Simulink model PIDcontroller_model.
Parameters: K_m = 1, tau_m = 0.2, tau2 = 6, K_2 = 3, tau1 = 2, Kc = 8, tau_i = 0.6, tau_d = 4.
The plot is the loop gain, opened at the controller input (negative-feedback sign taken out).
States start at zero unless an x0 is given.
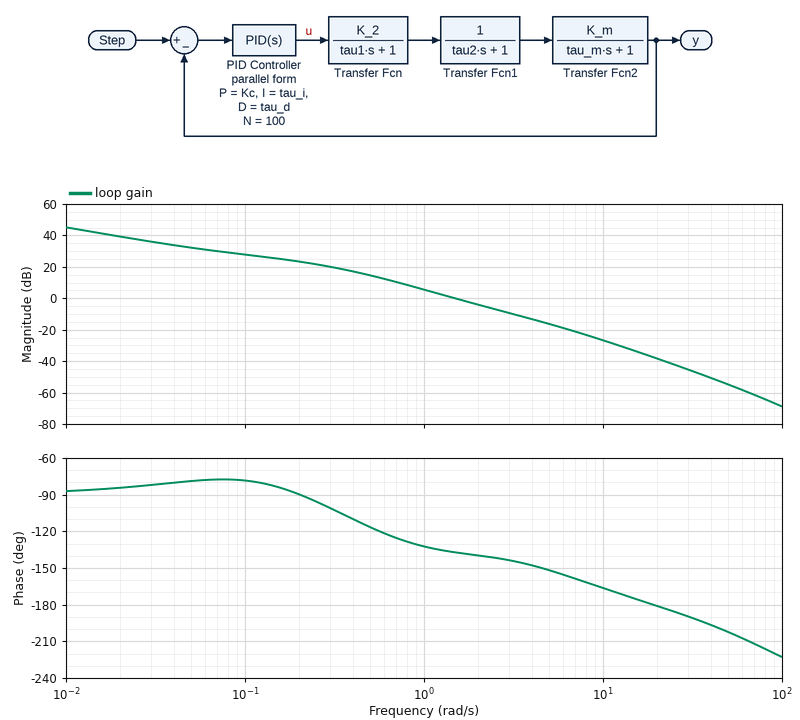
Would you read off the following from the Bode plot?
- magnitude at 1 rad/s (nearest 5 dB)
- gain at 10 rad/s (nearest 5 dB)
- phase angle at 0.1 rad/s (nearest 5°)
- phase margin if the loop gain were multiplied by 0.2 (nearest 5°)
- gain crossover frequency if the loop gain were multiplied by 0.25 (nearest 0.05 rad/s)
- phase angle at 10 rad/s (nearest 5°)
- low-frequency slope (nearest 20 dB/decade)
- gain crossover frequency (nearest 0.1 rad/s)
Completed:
5 dB
-25 dB
-80°
60°
0.60 rad/s
-165°
-20 dB/decade
1.5 rad/s
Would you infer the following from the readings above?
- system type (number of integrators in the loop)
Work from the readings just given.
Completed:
1
